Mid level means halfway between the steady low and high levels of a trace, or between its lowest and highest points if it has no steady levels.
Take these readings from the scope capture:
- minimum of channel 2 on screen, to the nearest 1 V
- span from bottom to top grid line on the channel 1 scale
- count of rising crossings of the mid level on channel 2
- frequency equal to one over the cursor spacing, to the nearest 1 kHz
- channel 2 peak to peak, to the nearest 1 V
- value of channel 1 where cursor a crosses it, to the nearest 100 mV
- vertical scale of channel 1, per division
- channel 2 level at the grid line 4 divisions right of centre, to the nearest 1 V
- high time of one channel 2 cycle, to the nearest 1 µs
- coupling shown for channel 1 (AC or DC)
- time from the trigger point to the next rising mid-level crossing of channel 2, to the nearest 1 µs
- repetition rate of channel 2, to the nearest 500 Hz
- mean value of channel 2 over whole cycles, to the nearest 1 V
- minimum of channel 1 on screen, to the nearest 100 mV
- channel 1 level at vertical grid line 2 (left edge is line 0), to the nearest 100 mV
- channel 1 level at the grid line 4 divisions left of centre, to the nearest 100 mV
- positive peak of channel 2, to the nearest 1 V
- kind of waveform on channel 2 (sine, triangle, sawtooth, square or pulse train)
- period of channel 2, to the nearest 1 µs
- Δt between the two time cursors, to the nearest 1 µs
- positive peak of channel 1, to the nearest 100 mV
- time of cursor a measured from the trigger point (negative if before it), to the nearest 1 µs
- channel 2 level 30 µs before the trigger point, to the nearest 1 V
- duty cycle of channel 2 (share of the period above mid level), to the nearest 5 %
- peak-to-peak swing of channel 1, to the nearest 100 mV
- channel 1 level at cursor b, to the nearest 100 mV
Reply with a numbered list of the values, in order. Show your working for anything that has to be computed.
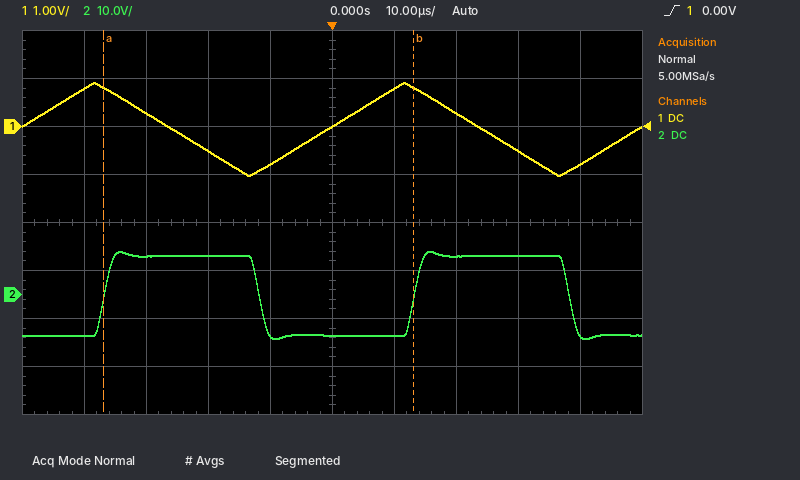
1. -9 V
2. 8 V
3. 2
4. 1 / 50 µs ≈ 20 kHz
5. 9 V − (-9 V) = 18 V
6. 800 mV
7. 1 V
8. -8 V
9. 25 µs
10. DC
11. 13 µs
12. 1 / 50 µs ≈ 20.0 kHz
13. -9 V + 0.5 × (9 V − (-9 V)) ≈ 0 V
14. -1.0 V
15. 300 mV
16. 800 mV
17. 9 V
18. square
19. 50 µs
20. 50 µs
21. 900 mV
22. -37 µs
23. 8 V
24. 25 µs / 50 µs ≈ 50 %
25. 900 mV − (-1.0 V) = 1.9 V
26. 800 mV
